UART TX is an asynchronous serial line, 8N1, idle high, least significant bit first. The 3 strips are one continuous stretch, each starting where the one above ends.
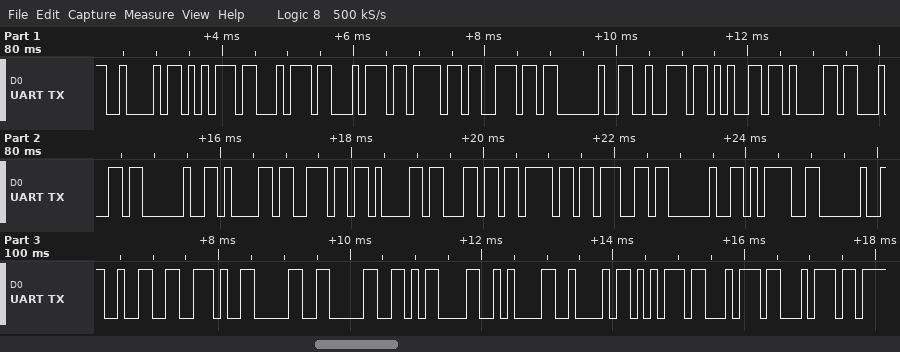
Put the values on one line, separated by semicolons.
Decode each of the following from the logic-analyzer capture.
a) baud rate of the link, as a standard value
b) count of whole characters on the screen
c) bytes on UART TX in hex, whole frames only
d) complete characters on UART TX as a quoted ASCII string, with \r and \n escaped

9600 baud; 31; 42 75 74 74 6F 6E 20 72 65 61 64 20 61 6E 61 6C 6F 67 20 3D 20 32 2E 30 30 0D 0A 42 75 74 74; "Button read analog = 2.00\r\nButt"
